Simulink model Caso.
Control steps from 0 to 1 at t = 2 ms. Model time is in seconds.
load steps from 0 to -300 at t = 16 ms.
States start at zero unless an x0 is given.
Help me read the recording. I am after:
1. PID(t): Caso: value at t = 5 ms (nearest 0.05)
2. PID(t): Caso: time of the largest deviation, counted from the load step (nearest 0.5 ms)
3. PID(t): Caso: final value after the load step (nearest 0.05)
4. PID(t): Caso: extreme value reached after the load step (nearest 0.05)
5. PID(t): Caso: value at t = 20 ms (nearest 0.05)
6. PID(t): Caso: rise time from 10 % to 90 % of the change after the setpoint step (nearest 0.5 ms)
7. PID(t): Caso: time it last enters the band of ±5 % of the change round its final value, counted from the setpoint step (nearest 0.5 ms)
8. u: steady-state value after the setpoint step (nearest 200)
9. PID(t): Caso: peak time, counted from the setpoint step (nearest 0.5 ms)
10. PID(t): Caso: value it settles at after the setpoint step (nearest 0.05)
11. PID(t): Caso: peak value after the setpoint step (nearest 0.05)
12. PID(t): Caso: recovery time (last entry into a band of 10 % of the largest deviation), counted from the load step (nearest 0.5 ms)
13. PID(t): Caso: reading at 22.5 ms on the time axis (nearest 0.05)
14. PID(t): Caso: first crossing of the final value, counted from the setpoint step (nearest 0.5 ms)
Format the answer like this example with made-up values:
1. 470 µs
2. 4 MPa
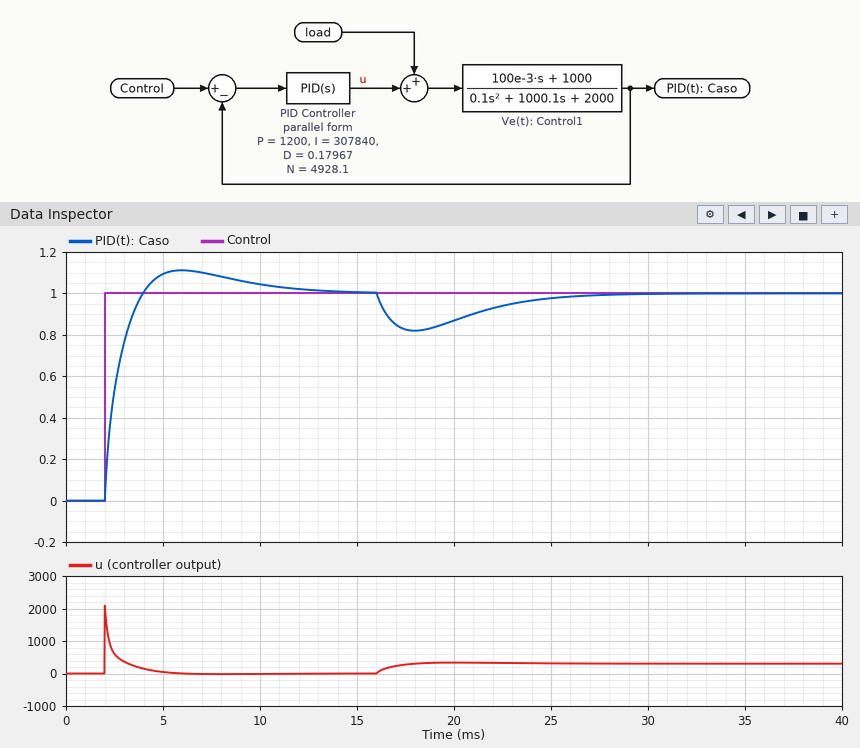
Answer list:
1. 1.10
2. 2.0 ms
3. 1.00
4. 0.80
5. 0.85
6. 1.5 ms
7. 7.5 ms
8. 0
9. 4.0 ms
10. 1.00
11. 1.10
12. 9.5 ms
13. 0.95
14. 2.0 ms
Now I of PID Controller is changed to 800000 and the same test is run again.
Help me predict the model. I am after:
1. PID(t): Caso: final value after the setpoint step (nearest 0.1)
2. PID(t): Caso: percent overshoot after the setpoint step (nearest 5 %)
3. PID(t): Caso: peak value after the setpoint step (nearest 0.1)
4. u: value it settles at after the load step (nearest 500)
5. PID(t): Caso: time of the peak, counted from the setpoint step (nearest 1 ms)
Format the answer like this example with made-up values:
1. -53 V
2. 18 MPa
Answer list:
1. 1.0
2. 20 %
3. 1.2
4. 500
5. 3 ms
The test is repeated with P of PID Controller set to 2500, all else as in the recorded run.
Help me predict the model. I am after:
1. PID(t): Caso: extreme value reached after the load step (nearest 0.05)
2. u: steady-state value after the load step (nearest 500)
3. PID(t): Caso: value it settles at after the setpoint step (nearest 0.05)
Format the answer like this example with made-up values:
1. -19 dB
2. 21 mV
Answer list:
1. 0.90
2. 500
3. 1.00
